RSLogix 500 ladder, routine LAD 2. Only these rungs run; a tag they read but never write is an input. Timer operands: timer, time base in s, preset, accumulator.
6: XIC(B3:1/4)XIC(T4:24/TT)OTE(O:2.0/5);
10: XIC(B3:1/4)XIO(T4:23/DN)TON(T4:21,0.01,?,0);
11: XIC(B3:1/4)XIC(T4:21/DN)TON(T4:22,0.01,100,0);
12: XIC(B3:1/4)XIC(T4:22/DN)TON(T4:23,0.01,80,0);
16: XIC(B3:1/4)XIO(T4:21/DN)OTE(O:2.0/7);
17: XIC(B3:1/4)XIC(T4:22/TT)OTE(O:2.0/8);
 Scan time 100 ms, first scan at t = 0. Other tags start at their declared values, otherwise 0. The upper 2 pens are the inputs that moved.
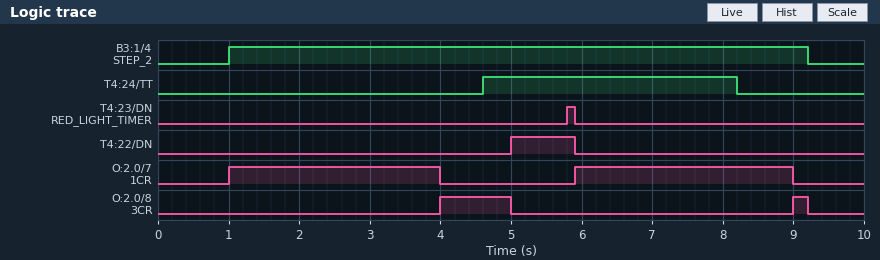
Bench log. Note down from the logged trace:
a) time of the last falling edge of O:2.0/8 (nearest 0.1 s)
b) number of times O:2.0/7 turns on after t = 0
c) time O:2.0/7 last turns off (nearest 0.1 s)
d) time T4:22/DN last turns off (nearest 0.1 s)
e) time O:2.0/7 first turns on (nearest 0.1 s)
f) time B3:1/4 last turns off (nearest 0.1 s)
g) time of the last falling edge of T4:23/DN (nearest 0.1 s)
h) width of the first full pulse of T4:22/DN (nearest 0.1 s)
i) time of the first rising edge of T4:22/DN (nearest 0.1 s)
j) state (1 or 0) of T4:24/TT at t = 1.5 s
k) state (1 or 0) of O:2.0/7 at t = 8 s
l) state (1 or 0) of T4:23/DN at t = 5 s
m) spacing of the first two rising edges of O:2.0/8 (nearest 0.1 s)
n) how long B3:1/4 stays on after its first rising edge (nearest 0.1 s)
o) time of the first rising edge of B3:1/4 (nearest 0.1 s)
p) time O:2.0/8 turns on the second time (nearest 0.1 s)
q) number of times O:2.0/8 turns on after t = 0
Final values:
9.2 s
2
9.0 s
5.9 s
1.0 s
9.2 s
5.9 s
0.9 s
5.0 s
0
1
0
5.0 s
8.2 s
1.0 s
9.0 s
2
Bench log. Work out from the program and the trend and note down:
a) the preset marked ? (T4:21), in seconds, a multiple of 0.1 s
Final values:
3.0 s
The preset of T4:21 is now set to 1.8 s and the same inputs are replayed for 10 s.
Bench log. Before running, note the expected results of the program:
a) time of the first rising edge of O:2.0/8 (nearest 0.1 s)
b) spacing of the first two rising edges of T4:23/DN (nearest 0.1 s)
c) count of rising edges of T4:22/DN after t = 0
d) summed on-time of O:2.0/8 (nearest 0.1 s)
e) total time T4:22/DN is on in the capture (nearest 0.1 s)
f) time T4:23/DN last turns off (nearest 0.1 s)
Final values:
2.8 s
3.8 s
2
2.0 s
1.8 s
8.5 s
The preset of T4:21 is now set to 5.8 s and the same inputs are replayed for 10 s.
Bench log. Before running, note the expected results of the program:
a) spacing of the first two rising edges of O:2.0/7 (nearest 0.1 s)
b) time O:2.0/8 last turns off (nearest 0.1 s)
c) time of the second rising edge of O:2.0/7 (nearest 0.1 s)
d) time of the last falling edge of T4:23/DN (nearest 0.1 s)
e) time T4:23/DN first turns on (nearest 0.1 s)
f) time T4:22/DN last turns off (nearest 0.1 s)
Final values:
7.7 s
7.8 s
8.7 s
8.7 s
8.6 s
8.7 s
